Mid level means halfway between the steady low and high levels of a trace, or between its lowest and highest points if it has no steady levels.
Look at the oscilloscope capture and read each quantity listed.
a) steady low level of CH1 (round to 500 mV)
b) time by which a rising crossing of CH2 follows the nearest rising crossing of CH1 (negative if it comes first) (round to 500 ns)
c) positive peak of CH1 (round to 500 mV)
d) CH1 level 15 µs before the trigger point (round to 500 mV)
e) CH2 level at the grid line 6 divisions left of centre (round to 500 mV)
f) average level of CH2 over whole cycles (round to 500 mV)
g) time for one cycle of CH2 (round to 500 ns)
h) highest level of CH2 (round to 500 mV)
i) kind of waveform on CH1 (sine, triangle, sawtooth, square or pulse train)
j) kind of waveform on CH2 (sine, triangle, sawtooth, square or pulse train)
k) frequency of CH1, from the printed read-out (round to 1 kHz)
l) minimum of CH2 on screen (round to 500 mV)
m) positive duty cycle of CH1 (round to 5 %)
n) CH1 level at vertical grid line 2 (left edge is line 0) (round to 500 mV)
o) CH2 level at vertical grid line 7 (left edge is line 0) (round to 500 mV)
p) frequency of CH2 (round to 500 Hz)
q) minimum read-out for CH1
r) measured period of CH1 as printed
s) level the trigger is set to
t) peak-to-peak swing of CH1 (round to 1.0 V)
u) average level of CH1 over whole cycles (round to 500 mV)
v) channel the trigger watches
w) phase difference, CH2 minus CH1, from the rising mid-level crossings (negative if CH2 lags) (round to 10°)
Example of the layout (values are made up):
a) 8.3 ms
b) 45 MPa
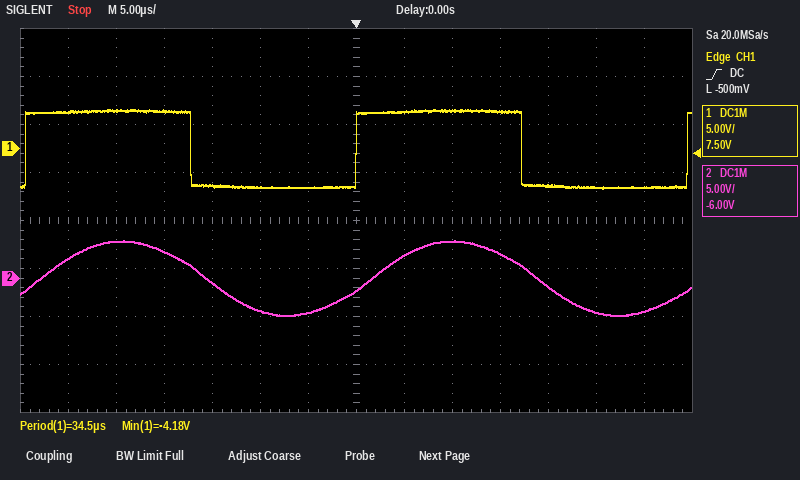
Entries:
a) -4.0 V
b) +1.5 µs
c) 4.0 V
d) -4.0 V
e) 2.0 V
f) 0.0 V
g) 34.5 µs
h) 4.0 V
i) square
j) sine
k) 29 kHz
l) -4.0 V
m) 50 %
n) 4.0 V
o) -1.5 V
p) 29.0 kHz
q) -4.18 V
r) 34.5 µs
s) -500 mV
t) 8.0 V
u) 0.0 V
v) CH1
w) -20°
